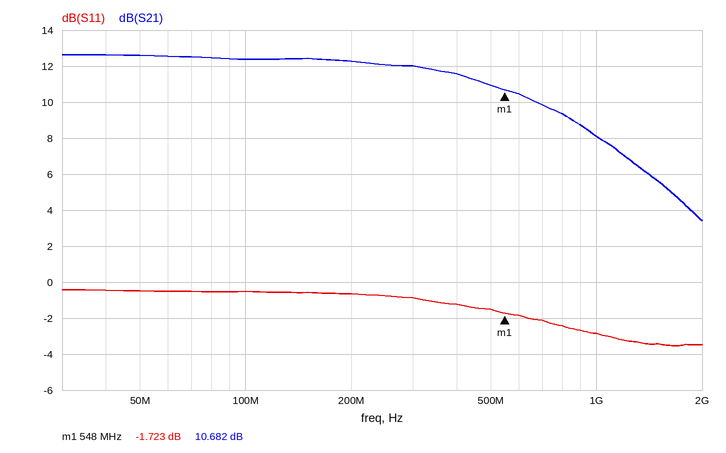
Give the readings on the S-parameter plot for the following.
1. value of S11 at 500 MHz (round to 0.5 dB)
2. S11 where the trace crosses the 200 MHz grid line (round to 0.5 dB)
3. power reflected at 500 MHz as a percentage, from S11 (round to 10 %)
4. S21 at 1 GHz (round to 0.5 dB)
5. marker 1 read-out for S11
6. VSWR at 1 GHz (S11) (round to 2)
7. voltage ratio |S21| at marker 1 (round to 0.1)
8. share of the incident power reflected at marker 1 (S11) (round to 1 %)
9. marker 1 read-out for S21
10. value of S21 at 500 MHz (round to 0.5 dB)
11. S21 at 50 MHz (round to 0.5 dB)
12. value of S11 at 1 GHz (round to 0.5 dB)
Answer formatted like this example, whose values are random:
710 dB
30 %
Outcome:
-1.5 dB
-0.5 dB
70 %
8.0 dB
-1.723 dB
6
3.4
67 %
10.682 dB
11.0 dB
12.5 dB
-3.0 dB
